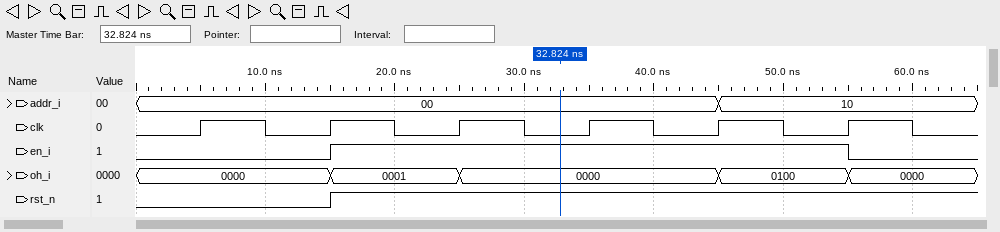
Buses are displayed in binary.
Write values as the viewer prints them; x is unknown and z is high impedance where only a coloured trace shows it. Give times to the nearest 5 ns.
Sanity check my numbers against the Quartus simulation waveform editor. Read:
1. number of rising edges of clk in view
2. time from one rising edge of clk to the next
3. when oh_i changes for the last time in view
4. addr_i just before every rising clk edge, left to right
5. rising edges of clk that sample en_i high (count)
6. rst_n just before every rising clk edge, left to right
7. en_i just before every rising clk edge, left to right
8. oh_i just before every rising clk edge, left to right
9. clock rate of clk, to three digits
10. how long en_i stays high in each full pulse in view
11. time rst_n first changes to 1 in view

6
10 ns
55 ns
00, 00, 00, 00, 00, 10
4
0 0 1 1 1 1
0 0 1 1 1 1
0000, 0000, 0001, 0000, 0000, 0100
100 MHz
40 ns
15 ns
